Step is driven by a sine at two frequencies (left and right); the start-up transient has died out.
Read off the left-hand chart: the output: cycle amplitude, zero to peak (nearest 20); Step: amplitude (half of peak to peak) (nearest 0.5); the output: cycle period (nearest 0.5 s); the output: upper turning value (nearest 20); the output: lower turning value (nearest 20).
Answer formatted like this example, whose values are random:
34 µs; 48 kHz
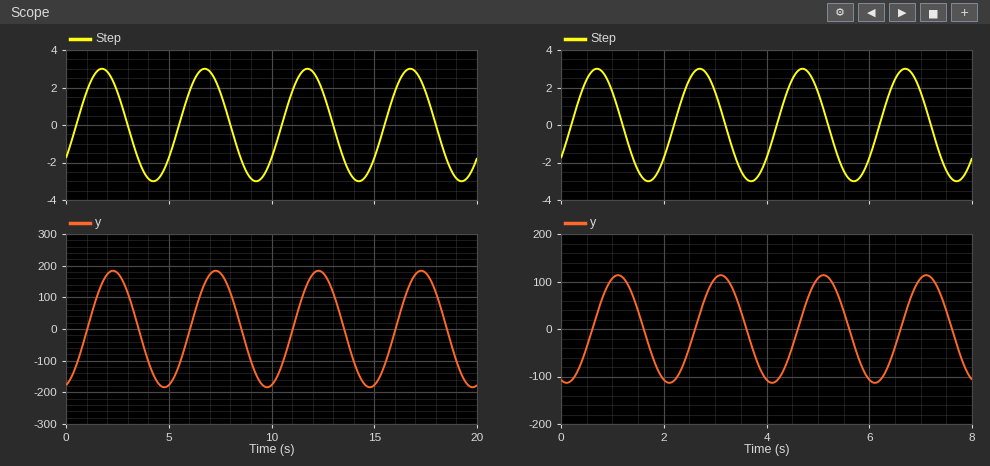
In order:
180; 3.0; 5.0 s; 180; -180
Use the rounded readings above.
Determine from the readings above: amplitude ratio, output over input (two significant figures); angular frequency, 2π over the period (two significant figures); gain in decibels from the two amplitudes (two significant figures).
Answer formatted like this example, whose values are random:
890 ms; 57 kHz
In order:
60; 1.3 rad/s; 36 dB
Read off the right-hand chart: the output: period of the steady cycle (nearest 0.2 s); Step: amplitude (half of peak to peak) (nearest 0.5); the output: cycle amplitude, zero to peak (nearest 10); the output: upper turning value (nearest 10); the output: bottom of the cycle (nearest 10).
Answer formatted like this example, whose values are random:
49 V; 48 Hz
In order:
2.0 s; 3.0; 110; 110; -110
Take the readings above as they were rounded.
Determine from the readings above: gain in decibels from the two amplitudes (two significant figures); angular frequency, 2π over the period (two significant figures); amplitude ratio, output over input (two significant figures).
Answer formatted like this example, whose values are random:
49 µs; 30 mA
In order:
31 dB; 3.1 rad/s; 37
